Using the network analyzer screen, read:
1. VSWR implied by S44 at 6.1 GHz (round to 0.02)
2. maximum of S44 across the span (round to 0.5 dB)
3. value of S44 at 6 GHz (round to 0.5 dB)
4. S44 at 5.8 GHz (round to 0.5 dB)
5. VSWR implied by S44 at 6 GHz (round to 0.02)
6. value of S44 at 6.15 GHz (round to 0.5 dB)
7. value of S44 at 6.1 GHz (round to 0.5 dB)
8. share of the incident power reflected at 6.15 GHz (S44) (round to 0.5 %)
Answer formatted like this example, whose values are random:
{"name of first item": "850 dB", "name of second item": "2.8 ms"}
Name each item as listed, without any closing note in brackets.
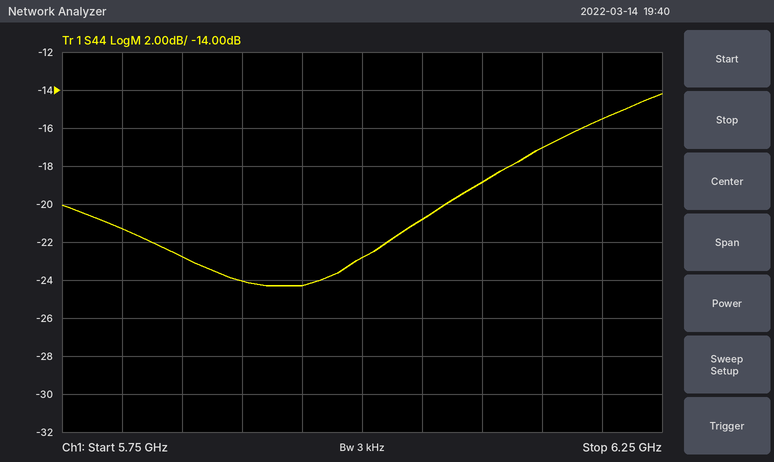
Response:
{"VSWR implied by S44 at 6.1 GHz": "1.26", "maximum of S44 across the span": "-14.0 dB", "value of S44 at 6 GHz": "-23.0 dB", "S44 at 5.8 GHz": "-21.5 dB", "VSWR implied by S44 at 6 GHz": "1.16", "value of S44 at 6.15 GHz": "-17.0 dB", "value of S44 at 6.1 GHz": "-19.0 dB", "share of the incident power reflected at 6.15 GHz (S44)": "2.0 %"}
